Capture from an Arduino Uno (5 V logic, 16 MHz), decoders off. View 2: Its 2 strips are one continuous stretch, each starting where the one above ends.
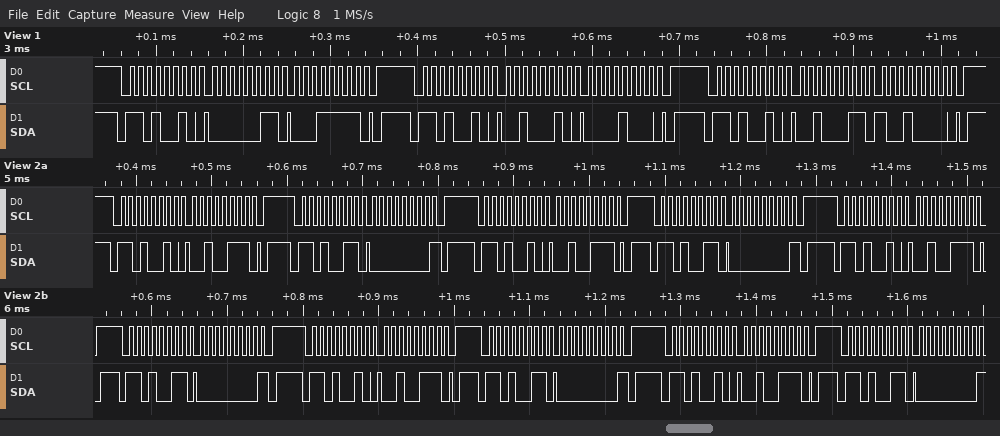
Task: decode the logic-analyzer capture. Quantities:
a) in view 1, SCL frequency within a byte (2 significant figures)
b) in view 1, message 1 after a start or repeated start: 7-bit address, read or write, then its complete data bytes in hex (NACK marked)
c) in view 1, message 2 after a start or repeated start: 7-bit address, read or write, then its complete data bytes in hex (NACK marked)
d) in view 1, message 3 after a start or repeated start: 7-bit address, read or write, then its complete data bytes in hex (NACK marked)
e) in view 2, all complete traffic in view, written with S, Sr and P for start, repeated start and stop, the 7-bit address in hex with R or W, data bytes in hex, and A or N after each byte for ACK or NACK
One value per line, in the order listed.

100 kHz
0x69 write: 03 1F
0x69 write: 22 08
0x69 write: 23 90
S 69W A 27 A P S 69R A 00 N P S 69W A 27 A P S 69R A 00 N P S 69W A 27 A P S 69R A 00 N P S 69W A 27 A P S 69R A 00 N P S 69W A 27 A P S 69R A 00 N
